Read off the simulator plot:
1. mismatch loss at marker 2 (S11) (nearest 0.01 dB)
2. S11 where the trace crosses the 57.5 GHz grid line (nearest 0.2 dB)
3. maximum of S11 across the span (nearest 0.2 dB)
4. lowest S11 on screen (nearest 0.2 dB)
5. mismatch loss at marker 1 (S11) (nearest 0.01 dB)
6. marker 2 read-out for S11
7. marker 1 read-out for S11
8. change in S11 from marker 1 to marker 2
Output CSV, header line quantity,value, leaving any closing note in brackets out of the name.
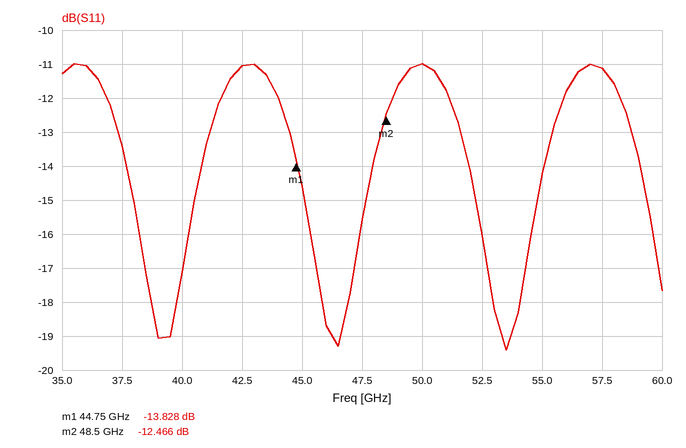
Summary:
quantity,value
mismatch loss at marker 2 (S11),0.25 dB
S11 where the trace crosses the 57.5 GHz grid line,-11.2 dB
maximum of S11 across the span,-11.0 dB
lowest S11 on screen,-19.4 dB
mismatch loss at marker 1 (S11),0.18 dB
marker 2 read-out for S11,-12.466 dB
marker 1 read-out for S11,-13.828 dB
change in S11 from marker 1 to marker 2,1.362 dB
